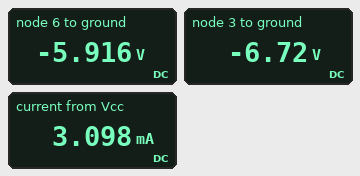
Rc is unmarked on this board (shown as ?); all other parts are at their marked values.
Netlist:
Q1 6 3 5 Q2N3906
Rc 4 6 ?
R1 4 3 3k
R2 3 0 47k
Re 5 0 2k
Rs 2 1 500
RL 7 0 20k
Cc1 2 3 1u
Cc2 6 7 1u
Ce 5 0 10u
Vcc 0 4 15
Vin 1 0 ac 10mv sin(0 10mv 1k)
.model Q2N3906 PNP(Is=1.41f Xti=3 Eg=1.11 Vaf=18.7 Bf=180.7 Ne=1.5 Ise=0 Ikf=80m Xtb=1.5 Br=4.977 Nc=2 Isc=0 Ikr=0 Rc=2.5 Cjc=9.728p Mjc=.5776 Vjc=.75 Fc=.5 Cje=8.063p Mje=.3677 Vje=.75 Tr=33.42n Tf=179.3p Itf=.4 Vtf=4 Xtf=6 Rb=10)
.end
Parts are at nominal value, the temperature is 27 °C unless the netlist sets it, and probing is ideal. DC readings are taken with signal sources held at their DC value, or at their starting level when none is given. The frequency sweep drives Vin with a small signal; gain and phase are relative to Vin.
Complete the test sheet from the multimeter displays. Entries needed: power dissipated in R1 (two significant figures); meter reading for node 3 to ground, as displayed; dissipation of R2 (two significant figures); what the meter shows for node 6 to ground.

23 mW
-6.72 V
960 µW
-5.916 V
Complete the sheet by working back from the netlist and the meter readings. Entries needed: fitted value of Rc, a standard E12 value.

27 kΩ
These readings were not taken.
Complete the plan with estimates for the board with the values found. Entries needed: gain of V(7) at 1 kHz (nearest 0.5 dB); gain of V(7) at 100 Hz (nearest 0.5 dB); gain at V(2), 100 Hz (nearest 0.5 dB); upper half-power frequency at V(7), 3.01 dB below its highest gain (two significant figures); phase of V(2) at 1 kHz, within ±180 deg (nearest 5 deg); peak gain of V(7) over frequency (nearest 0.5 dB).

-31.0 dB
-21.5 dB
-0.5 dB
370 Hz
-65 deg
-21.5 dB
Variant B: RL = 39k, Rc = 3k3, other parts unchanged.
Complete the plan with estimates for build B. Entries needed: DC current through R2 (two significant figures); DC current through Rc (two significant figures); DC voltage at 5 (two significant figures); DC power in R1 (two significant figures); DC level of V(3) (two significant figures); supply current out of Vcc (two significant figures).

190 µA
2.1 mA
-8.0 V
13 mW
-8.8 V
4.2 mA
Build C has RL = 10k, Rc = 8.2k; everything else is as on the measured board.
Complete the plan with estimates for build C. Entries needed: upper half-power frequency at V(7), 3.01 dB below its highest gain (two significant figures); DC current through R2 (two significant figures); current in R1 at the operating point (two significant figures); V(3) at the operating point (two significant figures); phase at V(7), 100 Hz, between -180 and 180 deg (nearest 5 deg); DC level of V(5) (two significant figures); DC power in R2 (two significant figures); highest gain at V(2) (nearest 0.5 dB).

380 Hz
160 µA
2.5 mA
-7.5 V
0 deg
-6.7 V
1.2 mW
0 dB
